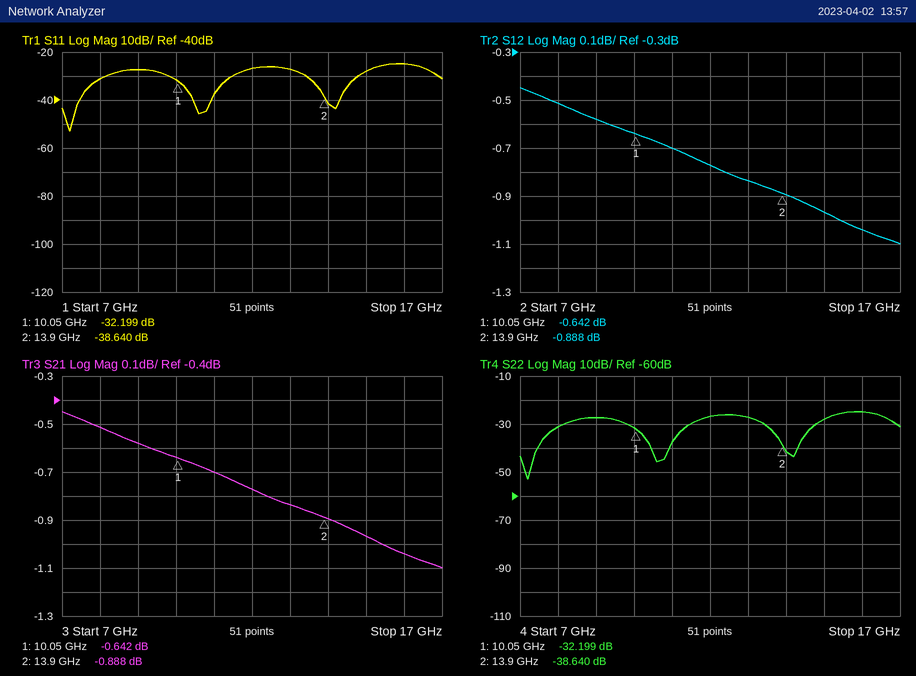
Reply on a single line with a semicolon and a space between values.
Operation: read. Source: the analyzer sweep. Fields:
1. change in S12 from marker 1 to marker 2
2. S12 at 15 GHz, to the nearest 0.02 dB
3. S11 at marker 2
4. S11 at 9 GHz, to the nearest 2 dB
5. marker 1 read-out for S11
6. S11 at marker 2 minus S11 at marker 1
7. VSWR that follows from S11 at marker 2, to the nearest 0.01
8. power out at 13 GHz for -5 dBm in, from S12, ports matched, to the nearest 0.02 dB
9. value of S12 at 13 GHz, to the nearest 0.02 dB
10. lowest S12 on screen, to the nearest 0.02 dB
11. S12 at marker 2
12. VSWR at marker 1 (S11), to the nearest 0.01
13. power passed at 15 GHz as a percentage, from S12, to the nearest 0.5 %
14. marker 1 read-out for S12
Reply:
-0.246 dB; -0.96 dB; -38.640 dB; -28 dB; -32.199 dB; -6.441 dB; 1.02; -5.84 dBm; -0.84 dB; -1.10 dB; -0.888 dB; 1.05; 80.0 %; -0.642 dB
